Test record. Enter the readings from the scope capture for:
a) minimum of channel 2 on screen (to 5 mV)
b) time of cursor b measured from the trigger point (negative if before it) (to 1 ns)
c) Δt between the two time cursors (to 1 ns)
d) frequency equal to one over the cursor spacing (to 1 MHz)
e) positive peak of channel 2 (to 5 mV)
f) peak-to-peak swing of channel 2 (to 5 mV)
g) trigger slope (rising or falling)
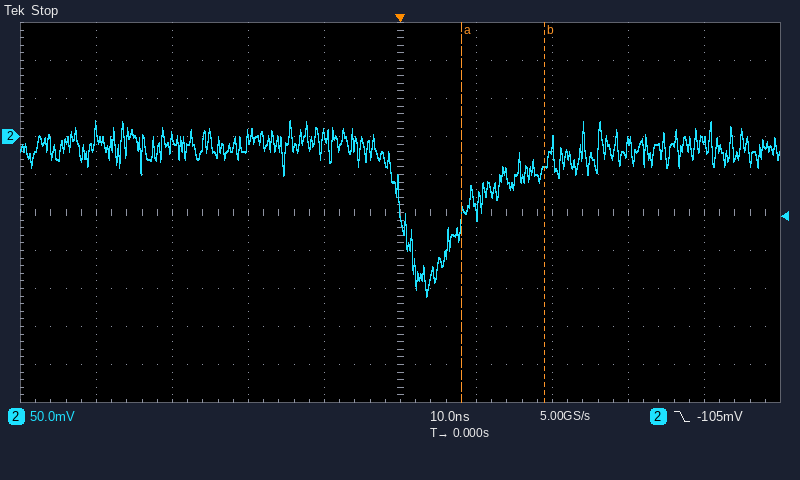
-210 mV
+19 ns
11 ns
91 MHz
20 mV
230 mV
falling
